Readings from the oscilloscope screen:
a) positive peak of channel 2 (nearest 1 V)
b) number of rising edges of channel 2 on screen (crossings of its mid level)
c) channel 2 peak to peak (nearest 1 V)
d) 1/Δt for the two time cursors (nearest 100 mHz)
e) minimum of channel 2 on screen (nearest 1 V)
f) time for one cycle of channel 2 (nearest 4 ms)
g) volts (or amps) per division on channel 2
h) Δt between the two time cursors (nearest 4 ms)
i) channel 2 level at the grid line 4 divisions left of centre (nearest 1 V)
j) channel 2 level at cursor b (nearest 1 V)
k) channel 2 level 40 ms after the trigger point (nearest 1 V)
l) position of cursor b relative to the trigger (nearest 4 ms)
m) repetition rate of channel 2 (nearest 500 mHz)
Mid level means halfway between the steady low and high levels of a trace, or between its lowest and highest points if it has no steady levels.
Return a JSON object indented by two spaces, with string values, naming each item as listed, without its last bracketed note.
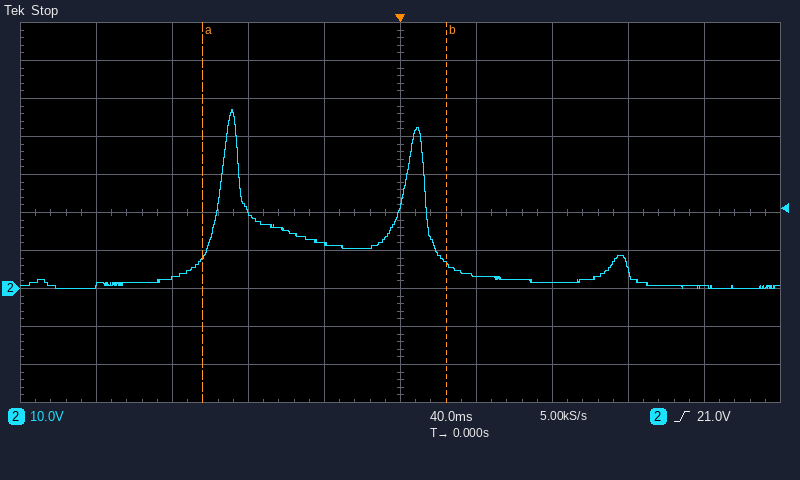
{
  "positive peak of channel 2": "47 V",
  "number of rising edges of channel 2 on screen": "2",
  "channel 2 peak to peak": "47 V",
  "1/Δt for the two time cursors": "7.8 Hz",
  "minimum of channel 2 on screen": "0 V",
  "time for one cycle of channel 2": "96 ms",
  "volts (or amps) per division on channel 2": "10 V",
  "Δt between the two time cursors": "128 ms",
  "channel 2 level at the grid line 4 divisions left of centre": "1 V",
  "channel 2 level at cursor b": "7 V",
  "channel 2 level 40 ms after the trigger point": "3 V",
  "position of cursor b relative to the trigger": "+24 ms",
  "repetition rate of channel 2": "10.5 Hz"
}
